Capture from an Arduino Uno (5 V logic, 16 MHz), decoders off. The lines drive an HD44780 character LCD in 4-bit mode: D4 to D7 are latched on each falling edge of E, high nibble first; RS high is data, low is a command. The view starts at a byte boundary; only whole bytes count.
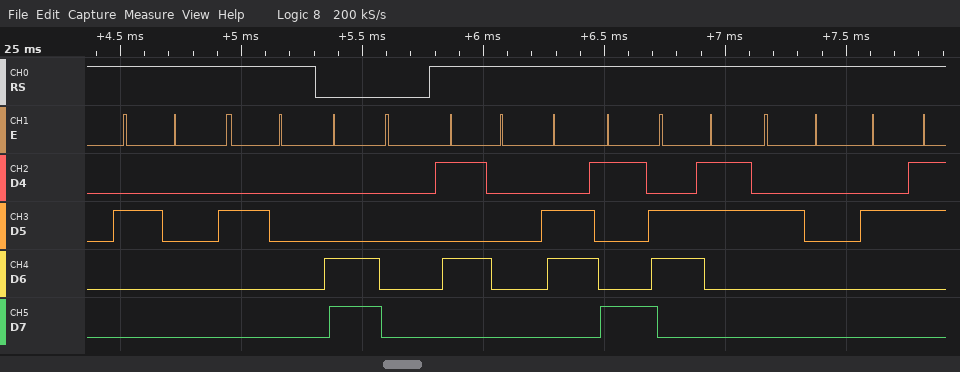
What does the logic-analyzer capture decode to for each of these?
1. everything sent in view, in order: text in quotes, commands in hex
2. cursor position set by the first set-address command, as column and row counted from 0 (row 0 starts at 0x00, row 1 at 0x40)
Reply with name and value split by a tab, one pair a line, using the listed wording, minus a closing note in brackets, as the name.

everything sent in view, in order: text in quotes, commands in hex	"  " 0xC0 "Pic #"
cursor position set by the first set-address command, as column and row counted from 0	column 0, row 1
